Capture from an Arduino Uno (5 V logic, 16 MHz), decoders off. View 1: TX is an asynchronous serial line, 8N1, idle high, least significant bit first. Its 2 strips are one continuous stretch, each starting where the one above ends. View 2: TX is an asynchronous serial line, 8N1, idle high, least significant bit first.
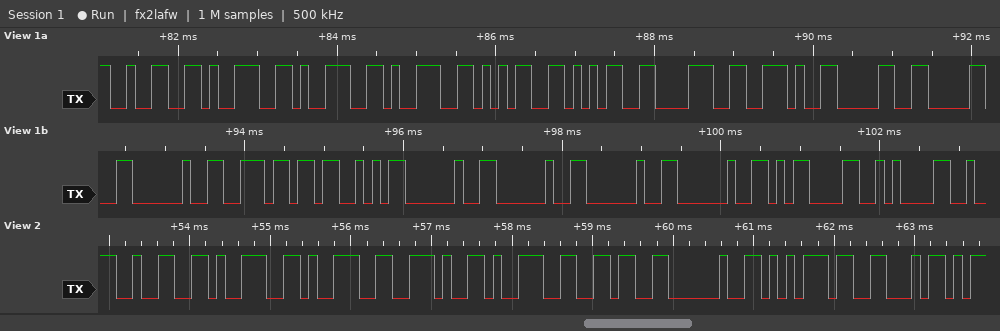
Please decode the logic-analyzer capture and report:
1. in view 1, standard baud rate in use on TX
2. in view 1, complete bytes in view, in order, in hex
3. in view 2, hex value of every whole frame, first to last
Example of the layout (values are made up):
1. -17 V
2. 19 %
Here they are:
1. 9600 baud
2. 32 39 39 39 35 35 38 2E 30 30 20 6E 53 20 20 20 20 0D 0A
3. 0x32 0x39 0x39 0x2E 0x39 0x36 0x20 0x75 0x46
